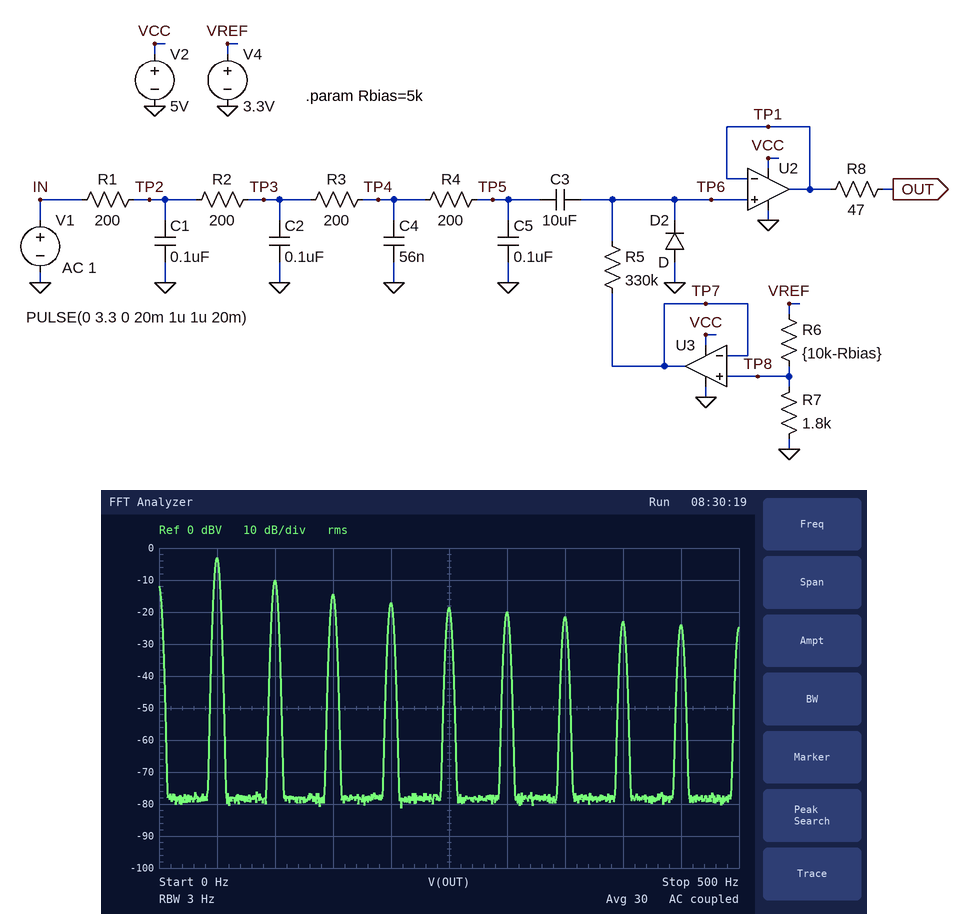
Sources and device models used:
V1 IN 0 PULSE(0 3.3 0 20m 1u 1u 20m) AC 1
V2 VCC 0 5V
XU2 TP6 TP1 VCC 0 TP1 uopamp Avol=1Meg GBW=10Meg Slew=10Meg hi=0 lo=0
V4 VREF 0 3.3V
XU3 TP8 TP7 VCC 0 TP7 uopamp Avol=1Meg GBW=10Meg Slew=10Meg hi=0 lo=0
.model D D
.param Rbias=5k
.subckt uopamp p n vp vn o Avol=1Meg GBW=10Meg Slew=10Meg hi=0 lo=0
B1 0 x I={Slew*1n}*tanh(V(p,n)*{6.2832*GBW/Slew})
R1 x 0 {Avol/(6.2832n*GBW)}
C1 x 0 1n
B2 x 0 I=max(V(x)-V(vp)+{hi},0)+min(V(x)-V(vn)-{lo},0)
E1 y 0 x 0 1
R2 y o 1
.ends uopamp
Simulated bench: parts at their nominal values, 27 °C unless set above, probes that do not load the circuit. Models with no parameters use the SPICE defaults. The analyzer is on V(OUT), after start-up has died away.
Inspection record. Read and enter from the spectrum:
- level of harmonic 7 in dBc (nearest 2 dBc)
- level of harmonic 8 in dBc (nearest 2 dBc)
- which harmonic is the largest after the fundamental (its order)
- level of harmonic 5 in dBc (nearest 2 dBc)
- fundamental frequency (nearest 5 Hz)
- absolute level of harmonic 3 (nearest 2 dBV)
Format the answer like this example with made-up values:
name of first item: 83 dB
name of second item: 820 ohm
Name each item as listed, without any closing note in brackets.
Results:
level of harmonic 7 in dBc: -18 dBc
level of harmonic 8 in dBc: -20 dBc
which harmonic is the largest after the fundamental: 2
level of harmonic 5 in dBc: -16 dBc
fundamental frequency: 50 Hz
absolute level of harmonic 3: -14 dBV
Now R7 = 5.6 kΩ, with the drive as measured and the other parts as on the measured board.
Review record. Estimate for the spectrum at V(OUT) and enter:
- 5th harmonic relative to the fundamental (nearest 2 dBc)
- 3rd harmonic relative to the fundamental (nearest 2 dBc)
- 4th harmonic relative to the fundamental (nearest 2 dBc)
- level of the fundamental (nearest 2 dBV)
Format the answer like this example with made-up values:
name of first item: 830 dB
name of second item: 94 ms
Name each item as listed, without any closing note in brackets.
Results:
5th harmonic relative to the fundamental: -14 dBc
3rd harmonic relative to the fundamental: -10 dBc
4th harmonic relative to the fundamental: -12 dBc
level of the fundamental: -2 dBV
